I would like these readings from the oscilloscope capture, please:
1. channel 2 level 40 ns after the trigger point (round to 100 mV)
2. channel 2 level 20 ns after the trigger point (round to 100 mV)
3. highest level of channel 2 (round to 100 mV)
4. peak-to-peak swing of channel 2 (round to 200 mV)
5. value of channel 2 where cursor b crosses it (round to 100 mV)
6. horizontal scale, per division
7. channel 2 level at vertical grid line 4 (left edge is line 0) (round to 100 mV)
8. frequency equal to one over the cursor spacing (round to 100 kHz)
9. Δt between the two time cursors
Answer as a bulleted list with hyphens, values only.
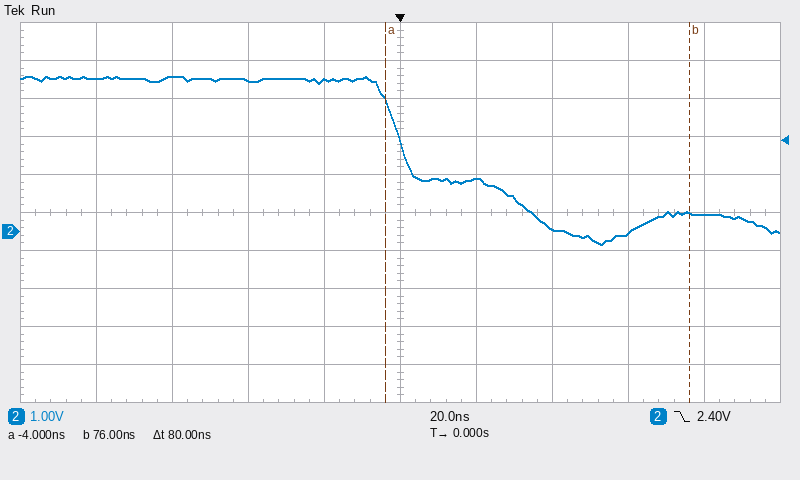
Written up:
- 100 mV
- 1.4 V
- 4.1 V
- 4.4 V
- 500 mV
- 20 ns
- 4.0 V
- 12.5 MHz
- 80 ns
